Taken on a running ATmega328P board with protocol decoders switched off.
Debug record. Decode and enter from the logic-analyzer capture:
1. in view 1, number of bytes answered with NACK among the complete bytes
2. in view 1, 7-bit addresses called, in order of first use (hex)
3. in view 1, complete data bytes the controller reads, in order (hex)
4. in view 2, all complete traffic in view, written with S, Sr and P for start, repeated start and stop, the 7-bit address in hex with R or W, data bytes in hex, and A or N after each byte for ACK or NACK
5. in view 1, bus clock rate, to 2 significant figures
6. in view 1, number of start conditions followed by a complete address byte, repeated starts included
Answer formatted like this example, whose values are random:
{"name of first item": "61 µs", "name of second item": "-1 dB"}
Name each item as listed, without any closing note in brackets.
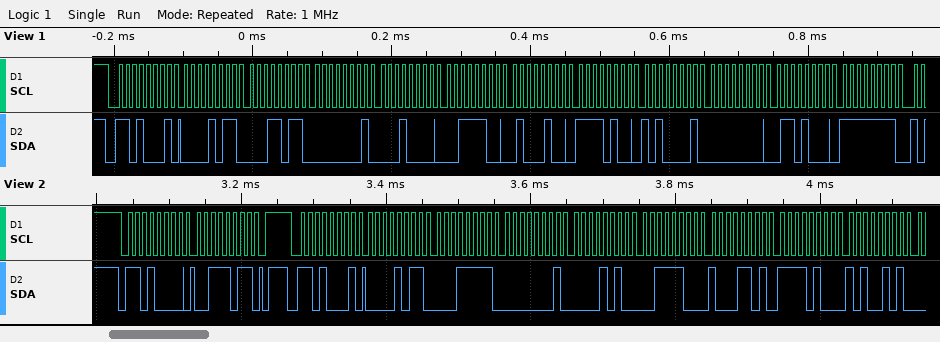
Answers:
{"in view 1, number of bytes answered with NACK among the complete bytes": "0", "in view 1, 7-bit addresses called, in order of first use": "0x68", "in view 1, complete data bytes the controller reads, in order": "0B 1B 01 10 3C 44 F4 A1 00 68 FF", "in view 2, all complete traffic in view, written with S, Sr and P for start, repeated start and stop, the 7-bit address in hex with R or W, data bytes in hex, and A or N after each byte for ACK or NACK": "S 68W A 3B A P S 68R A 0B A 1F A 01 A 0A A 3C A 8D A F4 A A5 A", "in view 1, bus clock rate, to 2 significant figures": "100 kHz", "in view 1, number of start conditions followed by a complete address byte, repeated starts included": "1"}
